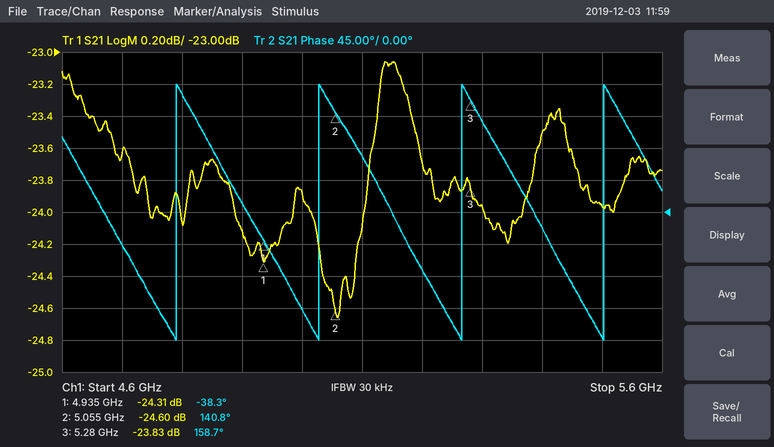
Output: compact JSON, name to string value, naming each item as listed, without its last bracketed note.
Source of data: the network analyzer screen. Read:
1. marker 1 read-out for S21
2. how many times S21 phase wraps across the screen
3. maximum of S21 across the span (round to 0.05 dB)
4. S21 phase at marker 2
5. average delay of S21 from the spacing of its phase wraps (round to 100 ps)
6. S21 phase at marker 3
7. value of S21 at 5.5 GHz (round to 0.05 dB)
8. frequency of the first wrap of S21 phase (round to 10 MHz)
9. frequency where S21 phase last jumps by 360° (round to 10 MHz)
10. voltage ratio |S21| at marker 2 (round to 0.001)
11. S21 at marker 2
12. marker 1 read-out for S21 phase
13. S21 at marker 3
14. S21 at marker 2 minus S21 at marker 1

{"marker 1 read-out for S21": "-24.31 dB", "how many times S21 phase wraps across the screen": "4", "maximum of S21 across the span": "-23.05 dB", "S21 phase at marker 2": "140.8°", "average delay of S21 from the spacing of its phase wraps": "4.2 ns", "S21 phase at marker 3": "158.7°", "value of S21 at 5.5 GHz": "-23.95 dB", "frequency of the first wrap of S21 phase": "4.79 GHz", "frequency where S21 phase last jumps by 360°": "5.50 GHz", "voltage ratio |S21| at marker 2": "0.059", "S21 at marker 2": "-24.60 dB", "marker 1 read-out for S21 phase": "-38.3°", "S21 at marker 3": "-23.83 dB", "S21 at marker 2 minus S21 at marker 1": "-0.29 dB"}
